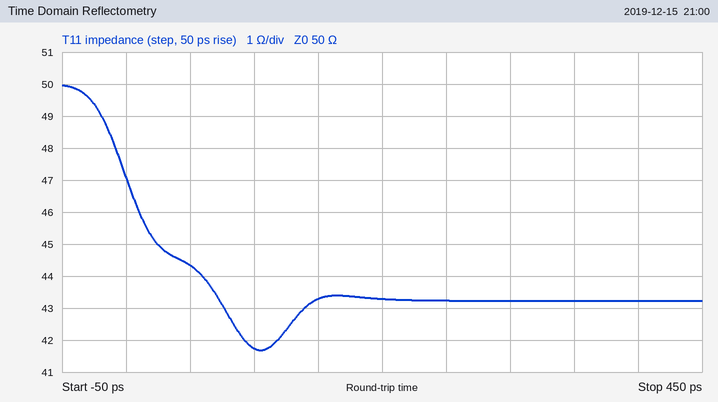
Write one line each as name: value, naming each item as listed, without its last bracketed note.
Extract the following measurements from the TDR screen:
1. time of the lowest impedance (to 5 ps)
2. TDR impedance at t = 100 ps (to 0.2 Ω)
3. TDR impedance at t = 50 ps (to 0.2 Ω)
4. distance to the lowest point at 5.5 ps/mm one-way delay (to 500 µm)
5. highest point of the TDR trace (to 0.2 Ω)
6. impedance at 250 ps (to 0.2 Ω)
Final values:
time of the lowest impedance: 105 ps
TDR impedance at t = 100 ps: 41.8 Ω
TDR impedance at t = 50 ps: 44.4 Ω
distance to the lowest point at 5.5 ps/mm one-way delay: 9.5 mm
highest point of the TDR trace: 50.0 Ω
impedance at 250 ps: 43.2 Ω
